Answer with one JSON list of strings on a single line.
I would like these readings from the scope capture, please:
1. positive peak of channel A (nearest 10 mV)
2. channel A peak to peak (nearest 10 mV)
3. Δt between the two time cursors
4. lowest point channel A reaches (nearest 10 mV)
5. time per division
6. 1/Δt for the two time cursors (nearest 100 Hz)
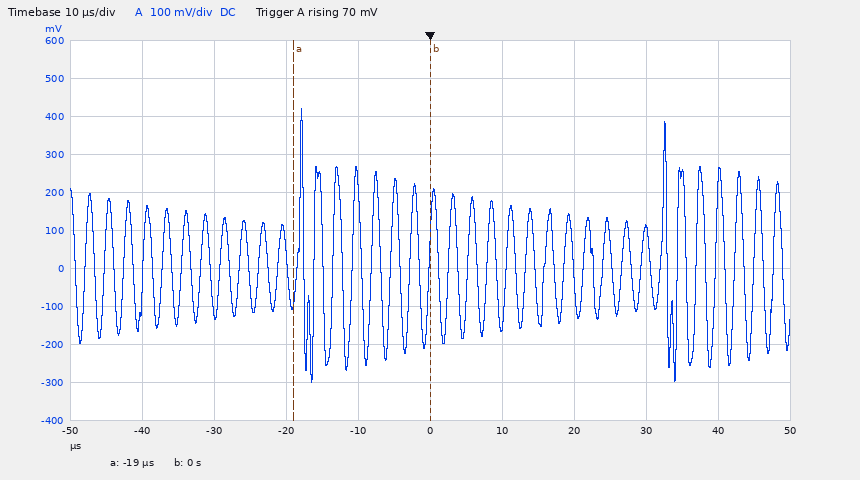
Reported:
["420 mV", "720 mV", "19 µs", "-300 mV", "10 µs", "52.6 kHz"]
